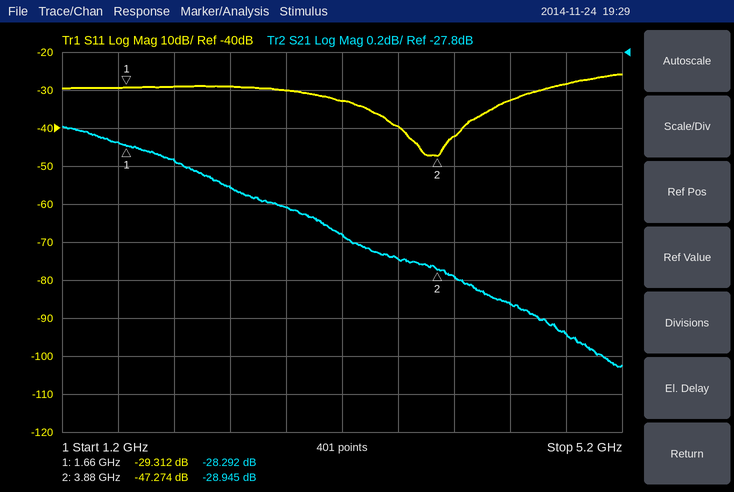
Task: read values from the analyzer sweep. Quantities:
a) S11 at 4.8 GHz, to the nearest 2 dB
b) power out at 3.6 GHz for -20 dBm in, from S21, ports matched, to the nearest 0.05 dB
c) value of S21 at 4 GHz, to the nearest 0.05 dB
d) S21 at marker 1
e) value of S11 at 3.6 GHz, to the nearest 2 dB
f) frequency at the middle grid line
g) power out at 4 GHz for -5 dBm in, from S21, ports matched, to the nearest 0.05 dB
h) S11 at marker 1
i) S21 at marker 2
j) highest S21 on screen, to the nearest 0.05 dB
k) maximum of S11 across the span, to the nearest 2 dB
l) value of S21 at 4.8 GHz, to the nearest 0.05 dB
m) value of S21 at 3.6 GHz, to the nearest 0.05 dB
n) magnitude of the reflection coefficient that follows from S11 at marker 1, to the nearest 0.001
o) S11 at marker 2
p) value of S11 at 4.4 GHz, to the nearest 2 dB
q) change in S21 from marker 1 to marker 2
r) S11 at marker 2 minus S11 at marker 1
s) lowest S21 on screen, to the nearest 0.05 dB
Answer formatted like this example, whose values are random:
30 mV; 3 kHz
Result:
-28 dB; -48.90 dBm; -29.00 dB; -28.292 dB; -40 dB; 3.2 GHz; -34.00 dBm; -29.312 dB; -28.945 dB; -28.20 dB; -26 dB; -29.30 dB; -28.90 dB; 0.034; -47.274 dB; -32 dB; -0.653 dB; -17.962 dB; -29.45 dB
